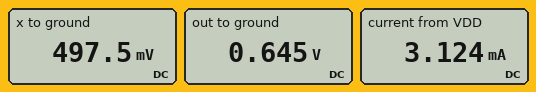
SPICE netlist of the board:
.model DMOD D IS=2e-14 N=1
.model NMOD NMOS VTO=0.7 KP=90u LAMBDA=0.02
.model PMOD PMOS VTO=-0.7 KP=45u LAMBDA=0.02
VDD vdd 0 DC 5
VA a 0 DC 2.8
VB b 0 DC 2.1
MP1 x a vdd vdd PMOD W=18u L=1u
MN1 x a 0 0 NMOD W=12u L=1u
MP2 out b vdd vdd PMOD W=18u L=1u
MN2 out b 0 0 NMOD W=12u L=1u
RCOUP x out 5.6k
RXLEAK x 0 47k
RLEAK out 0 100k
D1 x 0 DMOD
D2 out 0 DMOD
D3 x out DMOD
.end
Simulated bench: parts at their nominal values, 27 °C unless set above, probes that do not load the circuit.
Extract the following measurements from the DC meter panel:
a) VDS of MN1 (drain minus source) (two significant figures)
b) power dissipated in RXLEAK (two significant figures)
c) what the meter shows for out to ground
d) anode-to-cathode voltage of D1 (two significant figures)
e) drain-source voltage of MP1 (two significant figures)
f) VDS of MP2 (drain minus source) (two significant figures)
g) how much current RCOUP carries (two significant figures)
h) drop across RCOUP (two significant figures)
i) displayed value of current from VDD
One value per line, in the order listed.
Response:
500 mV
5.3 µW
0.645 V
500 mV
-4.5 V
-4.4 V
26 µA
150 mV
3.124 mA
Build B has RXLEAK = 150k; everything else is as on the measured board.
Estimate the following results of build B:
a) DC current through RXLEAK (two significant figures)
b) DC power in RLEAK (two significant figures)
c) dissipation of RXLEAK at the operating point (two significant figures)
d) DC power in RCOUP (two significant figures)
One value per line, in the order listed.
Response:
3.3 µA
4.2 µW
1.7 µW
3.7 µW
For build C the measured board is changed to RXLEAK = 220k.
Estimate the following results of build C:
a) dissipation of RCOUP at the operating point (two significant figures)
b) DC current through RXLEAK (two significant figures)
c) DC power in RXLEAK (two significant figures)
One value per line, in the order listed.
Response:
3.7 µW
2.3 µA
1.1 µW
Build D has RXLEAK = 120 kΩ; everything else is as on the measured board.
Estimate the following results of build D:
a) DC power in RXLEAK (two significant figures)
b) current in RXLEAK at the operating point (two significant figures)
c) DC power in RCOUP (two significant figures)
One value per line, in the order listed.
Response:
2.1 µW
4.2 µA
3.7 µW
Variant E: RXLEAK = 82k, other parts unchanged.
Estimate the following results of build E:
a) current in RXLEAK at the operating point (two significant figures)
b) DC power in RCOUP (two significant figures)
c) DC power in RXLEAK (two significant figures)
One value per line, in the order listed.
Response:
6.1 µA
3.8 µW
3.0 µW
